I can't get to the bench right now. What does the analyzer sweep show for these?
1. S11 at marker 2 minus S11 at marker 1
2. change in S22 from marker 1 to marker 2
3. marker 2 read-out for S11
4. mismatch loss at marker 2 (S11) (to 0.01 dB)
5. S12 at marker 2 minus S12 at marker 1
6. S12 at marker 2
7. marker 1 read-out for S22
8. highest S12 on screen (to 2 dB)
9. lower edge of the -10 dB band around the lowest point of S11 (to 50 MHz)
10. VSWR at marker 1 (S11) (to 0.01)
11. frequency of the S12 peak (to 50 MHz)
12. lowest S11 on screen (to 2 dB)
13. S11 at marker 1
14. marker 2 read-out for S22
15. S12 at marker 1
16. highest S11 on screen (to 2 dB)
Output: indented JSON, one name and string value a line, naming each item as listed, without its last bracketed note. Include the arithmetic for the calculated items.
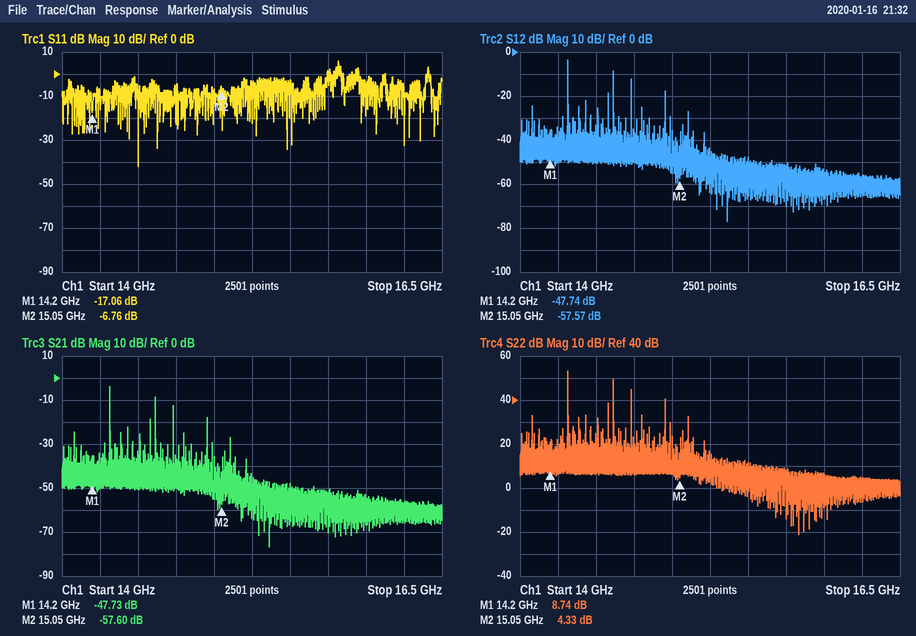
{
  "S11 at marker 2 minus S11 at marker 1": "-6.76 − (-17.06) = 10.30 dB",
  "change in S22 from marker 1 to marker 2": "4.33 − (8.74) = -4.41 dB",
  "marker 2 read-out for S11": "-6.76 dB",
  "mismatch loss at marker 2 (S11)": "−10 log10(1 − 10^(-6.76/10)) ≈ 1.03 dB",
  "S12 at marker 2 minus S12 at marker 1": "-57.57 − (-47.74) = -9.83 dB",
  "S12 at marker 2": "-57.57 dB",
  "marker 1 read-out for S22": "8.74 dB",
  "highest S12 on screen": "-4 dB",
  "lower edge of the -10 dB band around the lowest point of S11": "14.50 GHz",
  "VSWR at marker 1 (S11)": "(1 + 0.1403)/(1 − 0.1403) ≈ 1.33",
  "frequency of the S12 peak": "14.30 GHz",
  "lowest S11 on screen": "-42 dB",
  "S11 at marker 1": "-17.06 dB",
  "marker 2 read-out for S22": "4.33 dB",
  "S12 at marker 1": "-47.74 dB",
  "highest S11 on screen": "6 dB"
}
